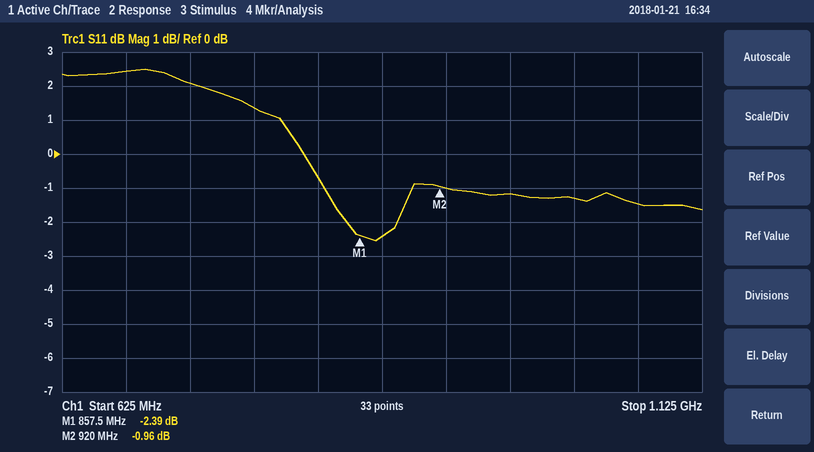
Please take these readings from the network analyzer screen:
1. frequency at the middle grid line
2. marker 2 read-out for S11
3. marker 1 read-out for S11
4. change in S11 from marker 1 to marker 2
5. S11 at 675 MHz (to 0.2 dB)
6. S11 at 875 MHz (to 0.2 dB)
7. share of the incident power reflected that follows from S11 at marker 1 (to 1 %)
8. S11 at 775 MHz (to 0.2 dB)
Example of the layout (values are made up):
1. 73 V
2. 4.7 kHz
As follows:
1. 875 MHz
2. -0.96 dB
3. -2.39 dB
4. 1.43 dB
5. 2.4 dB
6. -2.4 dB
7. 58 %
8. 1.4 dB
